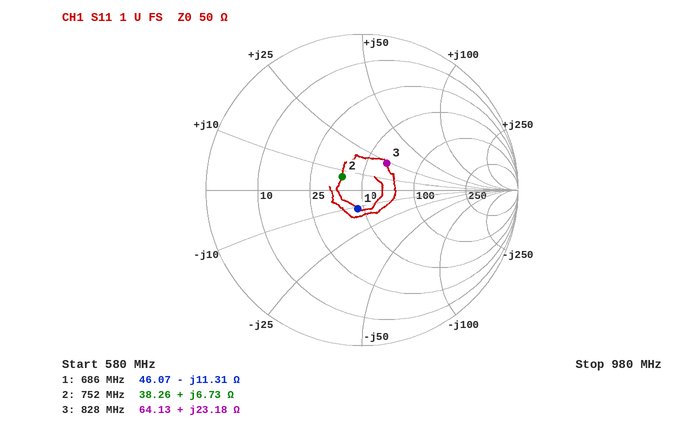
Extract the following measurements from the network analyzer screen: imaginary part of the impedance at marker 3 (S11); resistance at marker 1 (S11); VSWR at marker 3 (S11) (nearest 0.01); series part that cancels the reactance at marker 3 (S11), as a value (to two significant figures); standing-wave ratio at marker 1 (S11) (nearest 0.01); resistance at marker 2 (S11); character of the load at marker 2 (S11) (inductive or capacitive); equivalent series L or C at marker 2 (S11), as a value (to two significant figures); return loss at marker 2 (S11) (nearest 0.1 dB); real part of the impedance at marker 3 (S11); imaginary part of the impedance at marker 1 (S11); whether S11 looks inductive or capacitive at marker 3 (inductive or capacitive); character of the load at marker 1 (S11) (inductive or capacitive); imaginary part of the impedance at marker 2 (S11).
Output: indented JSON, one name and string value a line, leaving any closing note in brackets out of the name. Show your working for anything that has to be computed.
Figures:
{
  "imaginary part of the impedance at marker 3": "+23.18 Ω",
  "resistance at marker 1": "46.07 Ω",
  "VSWR at marker 3 (S11)": "1.61",
  "series part that cancels the reactance at marker 3 (S11), as a value": "C = 1/(2π × 828 MHz × 23.18 Ω) ≈ 8.3 pF",
  "standing-wave ratio at marker 1 (S11)": "1.28",
  "resistance at marker 2": "38.26 Ω",
  "character of the load at marker 2 (S11)": "inductive",
  "equivalent series L or C at marker 2 (S11), as a value": "L = 6.73 Ω/(2π × 752 MHz) ≈ 1.4 nH",
  "return loss at marker 2 (S11)": "16.3 dB",
  "real part of the impedance at marker 3": "64.13 Ω",
  "imaginary part of the impedance at marker 1": "-11.31 Ω",
  "whether S11 looks inductive or capacitive at marker 3": "inductive",
  "character of the load at marker 1 (S11)": "capacitive",
  "imaginary part of the impedance at marker 2": "+6.73 Ω"
}
